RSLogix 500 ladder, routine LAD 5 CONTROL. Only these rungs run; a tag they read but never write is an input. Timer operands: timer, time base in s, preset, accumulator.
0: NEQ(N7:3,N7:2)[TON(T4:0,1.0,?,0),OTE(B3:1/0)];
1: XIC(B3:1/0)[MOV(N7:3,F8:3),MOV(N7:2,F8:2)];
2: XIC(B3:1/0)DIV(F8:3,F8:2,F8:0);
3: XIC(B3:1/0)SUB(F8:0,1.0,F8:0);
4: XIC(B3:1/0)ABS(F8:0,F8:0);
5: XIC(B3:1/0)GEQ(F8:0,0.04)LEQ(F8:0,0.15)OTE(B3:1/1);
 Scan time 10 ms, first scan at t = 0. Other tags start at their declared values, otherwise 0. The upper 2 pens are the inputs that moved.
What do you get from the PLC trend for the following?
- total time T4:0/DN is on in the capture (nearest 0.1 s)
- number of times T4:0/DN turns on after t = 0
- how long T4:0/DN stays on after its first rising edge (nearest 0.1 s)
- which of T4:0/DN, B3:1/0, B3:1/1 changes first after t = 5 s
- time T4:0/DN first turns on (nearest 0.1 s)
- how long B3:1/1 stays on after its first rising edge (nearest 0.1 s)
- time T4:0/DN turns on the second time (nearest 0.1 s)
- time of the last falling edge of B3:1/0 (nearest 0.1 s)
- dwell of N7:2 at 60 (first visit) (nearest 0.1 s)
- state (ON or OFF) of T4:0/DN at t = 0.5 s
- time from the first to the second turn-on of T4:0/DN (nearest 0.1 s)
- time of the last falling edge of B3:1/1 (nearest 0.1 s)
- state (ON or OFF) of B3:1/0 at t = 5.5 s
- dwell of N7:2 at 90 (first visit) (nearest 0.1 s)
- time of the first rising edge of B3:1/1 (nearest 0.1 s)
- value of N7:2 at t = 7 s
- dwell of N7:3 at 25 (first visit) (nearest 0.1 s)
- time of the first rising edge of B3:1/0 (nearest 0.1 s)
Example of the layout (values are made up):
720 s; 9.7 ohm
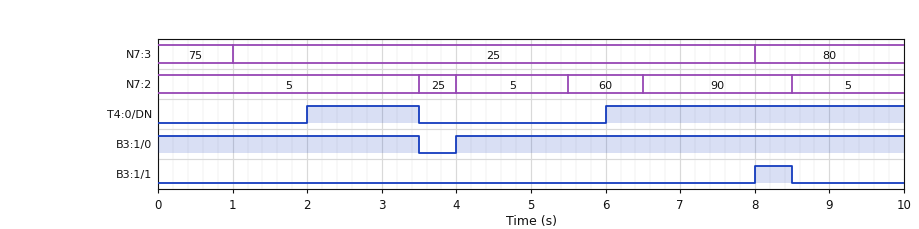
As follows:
5.5 s; 2; 1.5 s; T4:0/DN; 2.0 s; 0.5 s; 6.0 s; 3.5 s; 1.0 s; OFF; 4.0 s; 8.5 s; ON; 2.0 s; 8.0 s; 90; 7.0 s; 4.0 s
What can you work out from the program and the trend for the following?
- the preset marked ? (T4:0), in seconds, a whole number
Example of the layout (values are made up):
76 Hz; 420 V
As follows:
2 s
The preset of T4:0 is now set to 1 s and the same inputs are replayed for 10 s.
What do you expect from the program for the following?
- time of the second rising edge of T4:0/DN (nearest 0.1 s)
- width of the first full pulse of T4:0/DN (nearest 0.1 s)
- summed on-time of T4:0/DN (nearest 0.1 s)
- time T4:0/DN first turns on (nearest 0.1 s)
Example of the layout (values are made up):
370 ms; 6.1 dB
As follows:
5.0 s; 2.5 s; 7.5 s; 1.0 s
